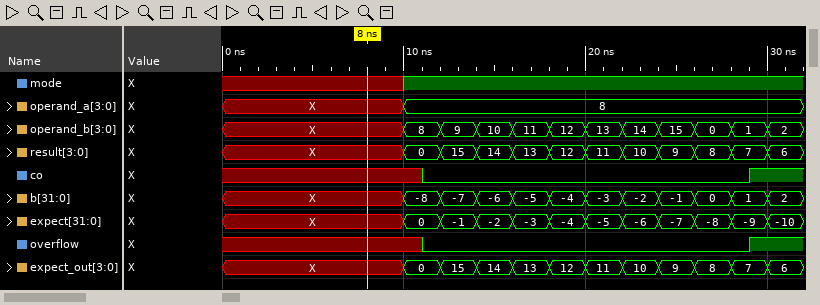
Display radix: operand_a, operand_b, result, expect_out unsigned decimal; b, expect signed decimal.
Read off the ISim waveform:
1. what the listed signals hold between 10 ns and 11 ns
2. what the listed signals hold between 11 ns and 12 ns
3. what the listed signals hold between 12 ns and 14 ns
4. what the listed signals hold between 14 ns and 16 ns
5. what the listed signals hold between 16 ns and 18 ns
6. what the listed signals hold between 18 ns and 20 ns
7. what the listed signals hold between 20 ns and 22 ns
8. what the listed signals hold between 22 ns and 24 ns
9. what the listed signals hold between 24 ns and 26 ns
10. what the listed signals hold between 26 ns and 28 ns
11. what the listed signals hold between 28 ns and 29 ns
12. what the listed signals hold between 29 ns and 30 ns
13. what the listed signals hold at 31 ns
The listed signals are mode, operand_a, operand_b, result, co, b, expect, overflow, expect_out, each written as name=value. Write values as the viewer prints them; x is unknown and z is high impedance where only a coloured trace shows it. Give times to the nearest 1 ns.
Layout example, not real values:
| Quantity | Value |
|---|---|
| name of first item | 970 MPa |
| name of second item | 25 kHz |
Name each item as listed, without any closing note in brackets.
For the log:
| Quantity | Value |
|---|---|
| what the listed signals hold between 10 ns and 11 ns | mode=1, operand_a=8, operand_b=8, result=0, co=x, b=-8, expect=0, overflow=x, expect_out=0 |
| what the listed signals hold between 11 ns and 12 ns | mode=1, operand_a=8, operand_b=8, result=0, co=0, b=-8, expect=0, overflow=0, expect_out=0 |
| what the listed signals hold between 12 ns and 14 ns | mode=1, operand_a=8, operand_b=9, result=15, co=0, b=-7, expect=-1, overflow=0, expect_out=15 |
| what the listed signals hold between 14 ns and 16 ns | mode=1, operand_a=8, operand_b=10, result=14, co=0, b=-6, expect=-2, overflow=0, expect_out=14 |
| what the listed signals hold between 16 ns and 18 ns | mode=1, operand_a=8, operand_b=11, result=13, co=0, b=-5, expect=-3, overflow=0, expect_out=13 |
| what the listed signals hold between 18 ns and 20 ns | mode=1, operand_a=8, operand_b=12, result=12, co=0, b=-4, expect=-4, overflow=0, expect_out=12 |
| what the listed signals hold between 20 ns and 22 ns | mode=1, operand_a=8, operand_b=13, result=11, co=0, b=-3, expect=-5, overflow=0, expect_out=11 |
| what the listed signals hold between 22 ns and 24 ns | mode=1, operand_a=8, operand_b=14, result=10, co=0, b=-2, expect=-6, overflow=0, expect_out=10 |
| what the listed signals hold between 24 ns and 26 ns | mode=1, operand_a=8, operand_b=15, result=9, co=0, b=-1, expect=-7, overflow=0, expect_out=9 |
| what the listed signals hold between 26 ns and 28 ns | mode=1, operand_a=8, operand_b=0, result=8, co=0, b=0, expect=-8, overflow=0, expect_out=8 |
| what the listed signals hold between 28 ns and 29 ns | mode=1, operand_a=8, operand_b=1, result=7, co=0, b=1, expect=-9, overflow=0, expect_out=7 |
| what the listed signals hold between 29 ns and 30 ns | mode=1, operand_a=8, operand_b=1, result=7, co=1, b=1, expect=-9, overflow=1, expect_out=7 |
| what the listed signals hold at 31 ns | mode=1, operand_a=8, operand_b=2, result=6, co=1, b=2, expect=-10, overflow=1, expect_out=6 |
